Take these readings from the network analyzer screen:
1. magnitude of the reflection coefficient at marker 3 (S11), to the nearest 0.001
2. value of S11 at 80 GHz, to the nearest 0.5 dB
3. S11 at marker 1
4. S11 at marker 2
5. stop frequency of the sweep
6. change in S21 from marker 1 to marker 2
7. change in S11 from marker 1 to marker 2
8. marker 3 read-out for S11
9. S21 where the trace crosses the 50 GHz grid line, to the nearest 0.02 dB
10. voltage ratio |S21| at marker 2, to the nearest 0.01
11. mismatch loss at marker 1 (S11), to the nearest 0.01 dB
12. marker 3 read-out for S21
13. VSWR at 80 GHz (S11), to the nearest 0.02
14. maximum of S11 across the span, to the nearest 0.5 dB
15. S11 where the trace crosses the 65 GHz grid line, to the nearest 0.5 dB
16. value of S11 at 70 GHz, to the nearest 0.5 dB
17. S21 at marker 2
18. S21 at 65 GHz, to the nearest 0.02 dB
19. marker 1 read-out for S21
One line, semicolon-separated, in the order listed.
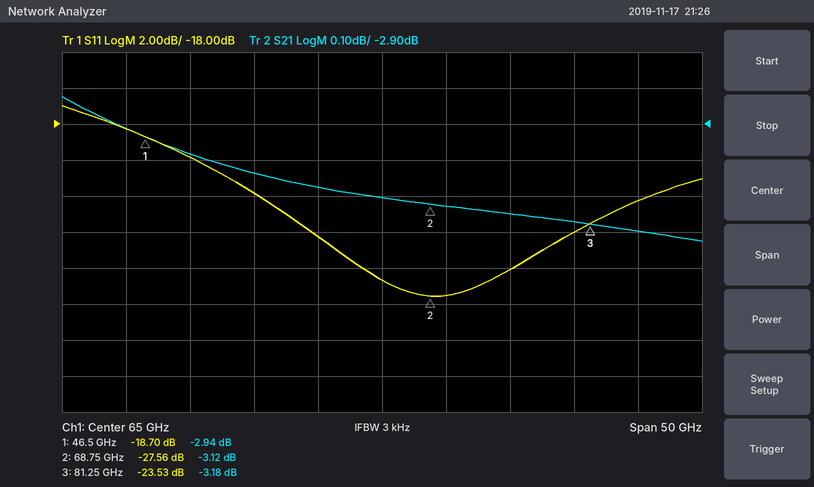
0.067; -24.0 dB; -18.70 dB; -27.56 dB; 90 GHz; -0.18 dB; -8.86 dB; -23.53 dB; -2.98 dB; 0.70; 0.06 dB; -3.18 dB; 1.14; -17.0 dB; -26.5 dB; -27.5 dB; -3.12 dB; -3.10 dB; -2.94 dB
